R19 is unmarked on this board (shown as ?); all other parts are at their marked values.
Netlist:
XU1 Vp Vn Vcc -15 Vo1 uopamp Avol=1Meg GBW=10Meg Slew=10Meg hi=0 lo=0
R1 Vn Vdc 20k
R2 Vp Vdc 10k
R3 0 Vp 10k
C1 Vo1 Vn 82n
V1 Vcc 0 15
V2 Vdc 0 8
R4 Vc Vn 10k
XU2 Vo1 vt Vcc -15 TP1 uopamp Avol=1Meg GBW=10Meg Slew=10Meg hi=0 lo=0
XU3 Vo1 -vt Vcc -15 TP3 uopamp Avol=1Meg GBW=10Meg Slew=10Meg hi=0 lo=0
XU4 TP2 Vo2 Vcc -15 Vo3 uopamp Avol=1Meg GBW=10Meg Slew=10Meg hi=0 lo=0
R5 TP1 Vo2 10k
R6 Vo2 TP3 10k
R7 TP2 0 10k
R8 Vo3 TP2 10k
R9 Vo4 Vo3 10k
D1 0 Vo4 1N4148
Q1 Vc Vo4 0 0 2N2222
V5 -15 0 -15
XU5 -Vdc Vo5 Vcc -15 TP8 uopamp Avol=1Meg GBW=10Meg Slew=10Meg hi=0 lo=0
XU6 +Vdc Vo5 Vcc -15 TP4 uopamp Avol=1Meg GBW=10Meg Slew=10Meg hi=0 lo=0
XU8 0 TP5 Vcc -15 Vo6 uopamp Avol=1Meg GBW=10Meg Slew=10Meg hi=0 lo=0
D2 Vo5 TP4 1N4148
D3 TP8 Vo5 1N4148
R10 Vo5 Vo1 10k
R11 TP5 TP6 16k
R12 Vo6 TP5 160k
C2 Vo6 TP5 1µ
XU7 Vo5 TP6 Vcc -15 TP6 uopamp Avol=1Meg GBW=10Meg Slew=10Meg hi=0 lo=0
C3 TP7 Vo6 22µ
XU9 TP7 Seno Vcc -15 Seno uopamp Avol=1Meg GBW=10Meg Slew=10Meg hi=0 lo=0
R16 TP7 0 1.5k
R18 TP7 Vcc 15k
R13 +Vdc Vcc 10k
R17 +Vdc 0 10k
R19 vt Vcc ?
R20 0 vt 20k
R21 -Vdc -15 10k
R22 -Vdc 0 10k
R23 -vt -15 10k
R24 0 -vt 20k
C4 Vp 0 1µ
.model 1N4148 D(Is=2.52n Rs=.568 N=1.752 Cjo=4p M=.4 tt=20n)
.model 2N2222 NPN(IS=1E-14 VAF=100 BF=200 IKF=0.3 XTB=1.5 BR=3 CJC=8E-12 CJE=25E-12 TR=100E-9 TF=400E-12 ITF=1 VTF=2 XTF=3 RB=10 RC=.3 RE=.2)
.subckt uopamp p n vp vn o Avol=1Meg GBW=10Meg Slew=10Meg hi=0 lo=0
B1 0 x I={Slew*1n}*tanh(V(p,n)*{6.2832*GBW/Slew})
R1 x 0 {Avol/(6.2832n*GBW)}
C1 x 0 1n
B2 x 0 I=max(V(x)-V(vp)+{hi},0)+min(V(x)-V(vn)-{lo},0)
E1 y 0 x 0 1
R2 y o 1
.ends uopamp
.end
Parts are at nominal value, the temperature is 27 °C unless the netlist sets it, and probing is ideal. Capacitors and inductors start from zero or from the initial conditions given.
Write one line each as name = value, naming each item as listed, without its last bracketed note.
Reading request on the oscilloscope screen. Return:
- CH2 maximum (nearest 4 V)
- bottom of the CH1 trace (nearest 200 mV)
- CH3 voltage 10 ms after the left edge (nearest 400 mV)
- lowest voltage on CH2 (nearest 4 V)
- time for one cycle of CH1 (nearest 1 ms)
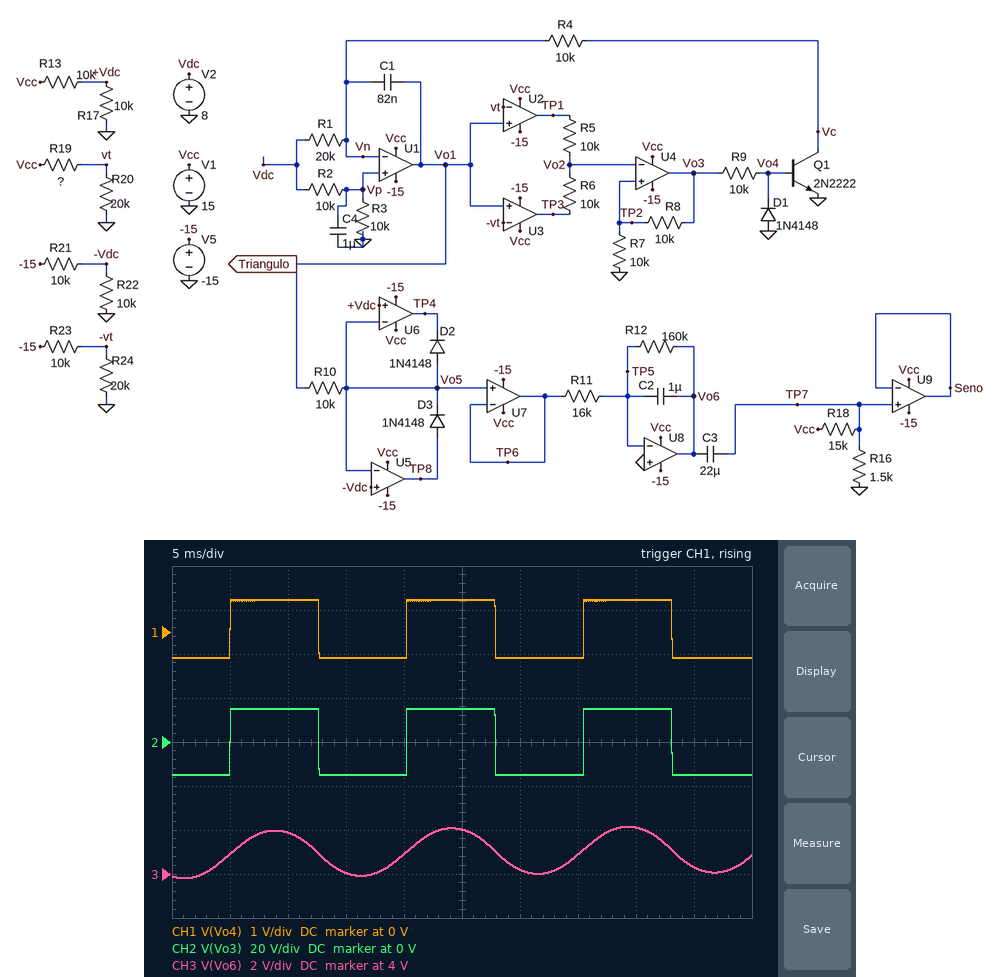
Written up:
CH2 maximum = 16 V
bottom of the CH1 trace = -600 mV
CH3 voltage 10 ms after the left edge = 6.0 V
lowest voltage on CH2 = -16 V
time for one cycle of CH1 = 15 ms
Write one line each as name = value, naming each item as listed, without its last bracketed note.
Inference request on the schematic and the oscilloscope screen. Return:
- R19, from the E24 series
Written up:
R19, from the E24 series = 15 kΩ
